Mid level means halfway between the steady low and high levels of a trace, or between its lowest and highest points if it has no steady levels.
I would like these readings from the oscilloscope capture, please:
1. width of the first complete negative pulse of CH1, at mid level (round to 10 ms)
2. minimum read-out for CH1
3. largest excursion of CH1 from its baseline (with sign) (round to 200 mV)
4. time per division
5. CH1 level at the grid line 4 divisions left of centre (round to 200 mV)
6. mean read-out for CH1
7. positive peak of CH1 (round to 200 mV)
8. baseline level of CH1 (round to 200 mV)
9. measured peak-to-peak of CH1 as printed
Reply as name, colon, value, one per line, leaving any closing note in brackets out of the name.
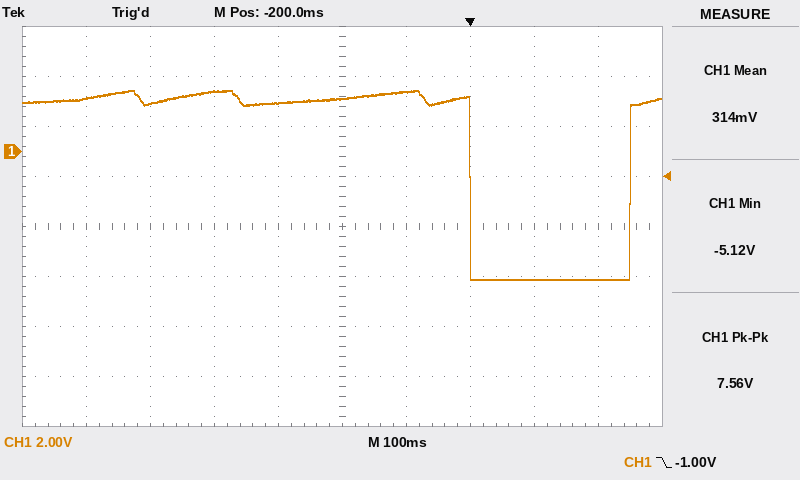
width of the first complete negative pulse of CH1, at mid level: 250 ms
minimum read-out for CH1: -5.12 V
largest excursion of CH1 from its baseline (with sign): -7.2 V
time per division: 100 ms
CH1 level at the grid line 4 divisions left of centre: 2.2 V
mean read-out for CH1: 314 mV
positive peak of CH1: 2.4 V
baseline level of CH1: 2.0 V
measured peak-to-peak of CH1 as printed: 7.56 V
